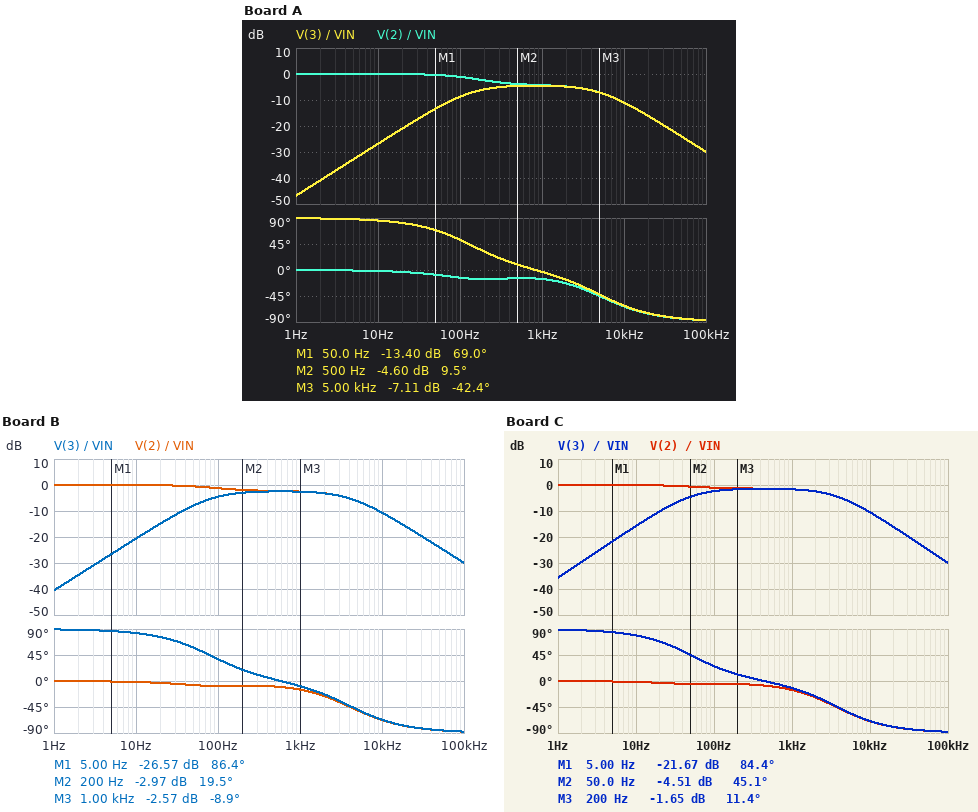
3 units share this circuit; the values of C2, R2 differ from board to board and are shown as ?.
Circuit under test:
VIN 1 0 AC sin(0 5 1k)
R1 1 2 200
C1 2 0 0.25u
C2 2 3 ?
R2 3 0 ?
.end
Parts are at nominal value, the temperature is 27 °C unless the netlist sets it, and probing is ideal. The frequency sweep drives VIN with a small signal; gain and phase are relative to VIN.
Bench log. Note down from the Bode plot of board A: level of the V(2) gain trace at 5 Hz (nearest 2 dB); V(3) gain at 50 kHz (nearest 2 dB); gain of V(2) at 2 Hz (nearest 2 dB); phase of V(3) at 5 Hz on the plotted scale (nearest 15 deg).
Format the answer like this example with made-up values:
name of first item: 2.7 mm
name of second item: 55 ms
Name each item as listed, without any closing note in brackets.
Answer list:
level of the V(2) gain trace at 5 Hz: 0 dB
V(3) gain at 50 kHz: -24 dB
gain of V(2) at 2 Hz: 0 dB
phase of V(3) at 5 Hz on the plotted scale: 90 deg
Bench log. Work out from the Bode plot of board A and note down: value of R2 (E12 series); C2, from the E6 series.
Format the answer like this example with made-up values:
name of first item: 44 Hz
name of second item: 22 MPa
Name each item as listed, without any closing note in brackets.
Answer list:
value of R2: 330 Ω
C2, from the E6 series: 2.2 µF
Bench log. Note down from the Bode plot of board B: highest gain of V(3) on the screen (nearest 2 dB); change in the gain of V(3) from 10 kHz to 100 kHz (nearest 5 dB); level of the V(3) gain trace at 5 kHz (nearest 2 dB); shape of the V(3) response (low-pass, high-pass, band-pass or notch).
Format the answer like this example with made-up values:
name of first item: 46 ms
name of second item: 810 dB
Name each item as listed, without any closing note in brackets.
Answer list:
highest gain of V(3) on the screen: -2 dB
change in the gain of V(3) from 10 kHz to 100 kHz: -20 dB
level of the V(3) gain trace at 5 kHz: -6 dB
shape of the V(3) response: band-pass
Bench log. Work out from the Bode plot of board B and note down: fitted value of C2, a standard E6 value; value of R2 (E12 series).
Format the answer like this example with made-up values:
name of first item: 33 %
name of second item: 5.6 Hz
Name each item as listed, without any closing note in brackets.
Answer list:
fitted value of C2, a standard E6 value: 2.2 µF
value of R2: 680 Ω
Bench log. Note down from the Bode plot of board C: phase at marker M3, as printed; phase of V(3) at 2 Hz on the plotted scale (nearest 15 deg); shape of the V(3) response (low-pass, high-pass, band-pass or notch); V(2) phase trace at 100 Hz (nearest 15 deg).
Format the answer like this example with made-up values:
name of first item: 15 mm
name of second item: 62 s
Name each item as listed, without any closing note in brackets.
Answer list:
phase at marker M3, as printed: 11.4 deg
phase of V(3) at 2 Hz on the plotted scale: 90 deg
shape of the V(3) response: band-pass
V(2) phase trace at 100 Hz: 0 deg
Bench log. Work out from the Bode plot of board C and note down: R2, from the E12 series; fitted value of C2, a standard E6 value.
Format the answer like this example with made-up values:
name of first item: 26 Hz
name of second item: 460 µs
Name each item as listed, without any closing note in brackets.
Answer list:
R2, from the E12 series: 1.2 kΩ
fitted value of C2, a standard E6 value: 2.2 µF
